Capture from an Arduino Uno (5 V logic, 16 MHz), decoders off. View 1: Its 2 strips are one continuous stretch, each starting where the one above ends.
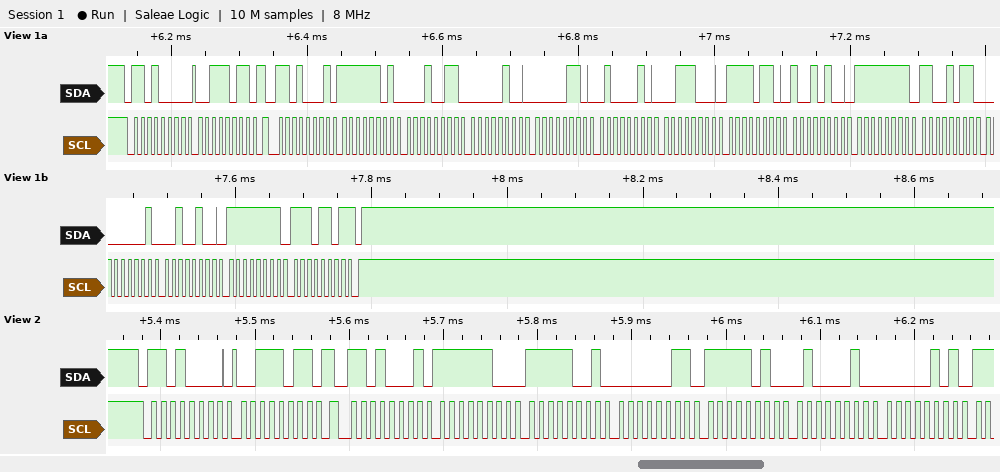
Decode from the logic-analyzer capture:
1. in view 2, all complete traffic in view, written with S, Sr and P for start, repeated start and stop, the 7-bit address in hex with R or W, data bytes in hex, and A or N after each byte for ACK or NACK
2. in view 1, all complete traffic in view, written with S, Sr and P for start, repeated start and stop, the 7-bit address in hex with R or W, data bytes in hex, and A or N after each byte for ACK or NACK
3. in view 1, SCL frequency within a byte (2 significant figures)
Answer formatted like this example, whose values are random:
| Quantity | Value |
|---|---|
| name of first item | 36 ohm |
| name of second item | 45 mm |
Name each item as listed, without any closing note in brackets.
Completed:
| Quantity | Value |
|---|---|
| in view 2, all complete traffic in view, written with S, Sr and P for start, repeated start and stop, the 7-bit address in hex with R or W, data bytes in hex, and A or N after each byte for ACK or NACK | S 68W A 3B A Sr 68R A FC A F9 A 03 A FA A 42 A 05 A |
| in view 1, all complete traffic in view, written with S, Sr and P for start, repeated start and stop, the 7-bit address in hex with R or W, data bytes in hex, and A or N after each byte for ACK or NACK | S 68W A 3B A Sr 68R A FD A 13 A 04 A 06 A 42 A 38 A F6 A 94 A FF A CB A 01 A 24 A FF A ED N P |
| in view 1, SCL frequency within a byte | 100 kHz |
